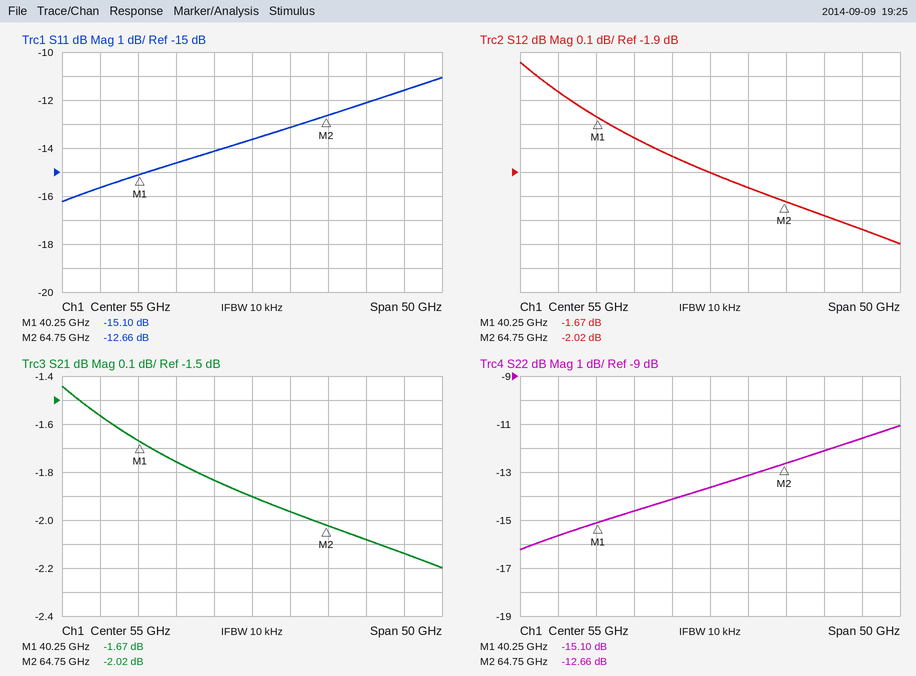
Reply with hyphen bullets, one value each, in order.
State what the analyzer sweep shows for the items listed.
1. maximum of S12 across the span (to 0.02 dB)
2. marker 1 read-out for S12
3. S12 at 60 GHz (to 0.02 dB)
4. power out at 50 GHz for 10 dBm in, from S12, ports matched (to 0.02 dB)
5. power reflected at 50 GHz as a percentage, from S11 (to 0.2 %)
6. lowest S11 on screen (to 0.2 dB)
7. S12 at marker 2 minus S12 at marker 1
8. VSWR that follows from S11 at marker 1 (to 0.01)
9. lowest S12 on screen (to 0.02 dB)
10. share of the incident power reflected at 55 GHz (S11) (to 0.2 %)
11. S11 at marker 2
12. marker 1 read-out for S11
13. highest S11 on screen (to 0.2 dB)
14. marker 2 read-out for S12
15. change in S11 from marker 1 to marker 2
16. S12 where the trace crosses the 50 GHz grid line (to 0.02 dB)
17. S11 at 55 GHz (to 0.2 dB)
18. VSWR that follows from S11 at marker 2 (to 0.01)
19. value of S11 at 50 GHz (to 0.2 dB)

- -1.44 dB
- -1.67 dB
- -1.96 dB
- 8.16 dBm
- 3.8 %
- -16.2 dB
- -0.35 dB
- 1.43
- -2.20 dB
- 4.4 %
- -12.66 dB
- -15.10 dB
- -11.0 dB
- -2.02 dB
- 2.44 dB
- -1.84 dB
- -13.6 dB
- 1.61
- -14.2 dB
